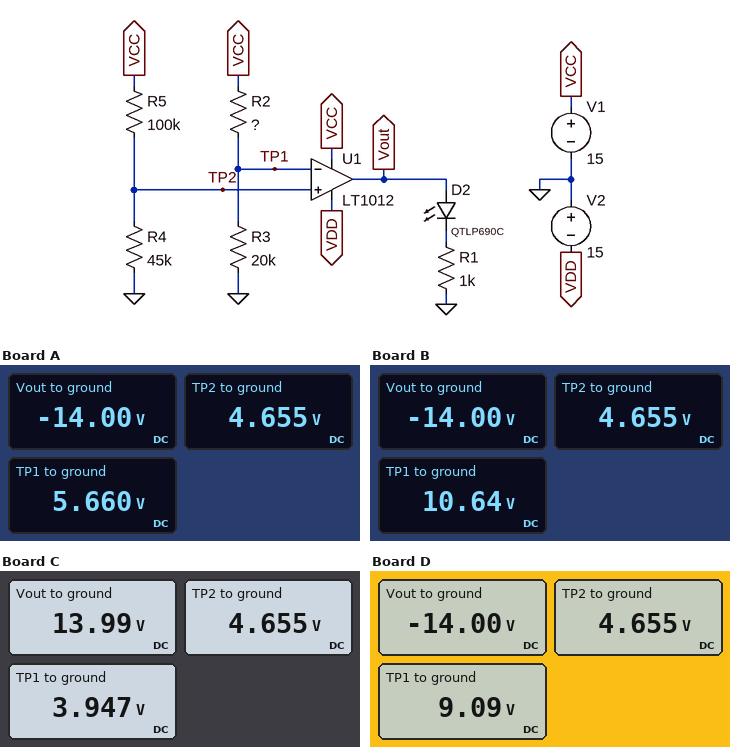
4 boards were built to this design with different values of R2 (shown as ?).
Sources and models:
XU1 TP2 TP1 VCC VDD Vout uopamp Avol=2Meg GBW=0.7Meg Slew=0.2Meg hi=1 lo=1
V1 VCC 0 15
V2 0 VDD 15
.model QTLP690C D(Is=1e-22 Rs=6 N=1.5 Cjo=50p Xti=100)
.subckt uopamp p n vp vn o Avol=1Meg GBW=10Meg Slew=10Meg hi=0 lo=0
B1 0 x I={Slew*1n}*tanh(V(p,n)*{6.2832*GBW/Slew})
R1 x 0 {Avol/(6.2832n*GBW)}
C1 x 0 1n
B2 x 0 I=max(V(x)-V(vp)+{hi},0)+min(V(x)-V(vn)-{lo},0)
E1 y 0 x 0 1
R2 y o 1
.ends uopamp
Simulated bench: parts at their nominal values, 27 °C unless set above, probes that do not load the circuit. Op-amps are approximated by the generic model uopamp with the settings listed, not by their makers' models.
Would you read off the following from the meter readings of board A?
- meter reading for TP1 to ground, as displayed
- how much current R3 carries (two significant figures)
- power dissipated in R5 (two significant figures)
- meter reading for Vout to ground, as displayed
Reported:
5.660 V
280 µA
1.1 mW
-14.00 V
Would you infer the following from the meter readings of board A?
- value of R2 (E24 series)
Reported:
33 kΩ
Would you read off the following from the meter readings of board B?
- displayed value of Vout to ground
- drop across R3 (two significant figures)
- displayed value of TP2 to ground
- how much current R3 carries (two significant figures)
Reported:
-14.00 V
11 V
4.655 V
530 µA
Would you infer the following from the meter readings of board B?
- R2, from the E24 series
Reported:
8.2 kΩ
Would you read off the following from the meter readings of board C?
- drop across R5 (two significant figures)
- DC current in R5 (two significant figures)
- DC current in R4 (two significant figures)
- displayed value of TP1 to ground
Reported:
10 V
100 µA
100 µA
3.947 V
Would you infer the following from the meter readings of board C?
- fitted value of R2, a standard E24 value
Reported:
56 kΩ
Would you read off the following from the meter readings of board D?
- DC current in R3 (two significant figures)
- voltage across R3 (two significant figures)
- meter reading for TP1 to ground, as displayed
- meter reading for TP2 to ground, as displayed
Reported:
450 µA
9.1 V
9.09 V
4.655 V
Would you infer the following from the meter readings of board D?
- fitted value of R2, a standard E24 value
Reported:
13 kΩ
